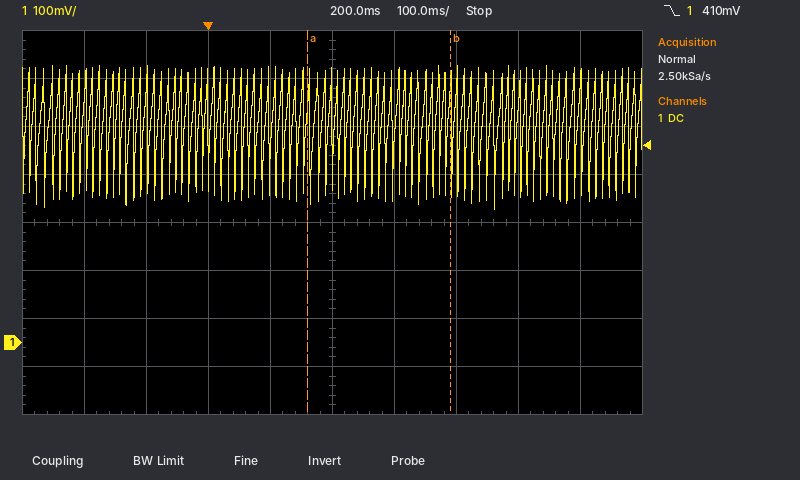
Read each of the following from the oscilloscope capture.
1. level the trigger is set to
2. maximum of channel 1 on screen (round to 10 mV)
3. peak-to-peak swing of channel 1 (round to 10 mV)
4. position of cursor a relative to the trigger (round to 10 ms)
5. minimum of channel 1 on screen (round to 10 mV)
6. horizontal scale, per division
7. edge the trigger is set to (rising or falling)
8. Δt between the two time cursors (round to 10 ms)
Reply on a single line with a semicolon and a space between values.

410 mV; 580 mV; 300 mV; +160 ms; 280 mV; 100 ms; falling; 230 ms
